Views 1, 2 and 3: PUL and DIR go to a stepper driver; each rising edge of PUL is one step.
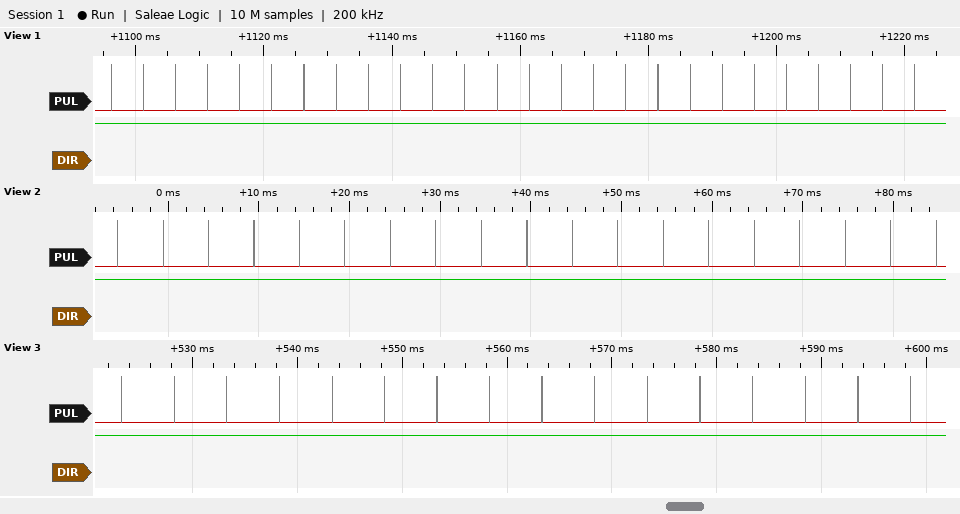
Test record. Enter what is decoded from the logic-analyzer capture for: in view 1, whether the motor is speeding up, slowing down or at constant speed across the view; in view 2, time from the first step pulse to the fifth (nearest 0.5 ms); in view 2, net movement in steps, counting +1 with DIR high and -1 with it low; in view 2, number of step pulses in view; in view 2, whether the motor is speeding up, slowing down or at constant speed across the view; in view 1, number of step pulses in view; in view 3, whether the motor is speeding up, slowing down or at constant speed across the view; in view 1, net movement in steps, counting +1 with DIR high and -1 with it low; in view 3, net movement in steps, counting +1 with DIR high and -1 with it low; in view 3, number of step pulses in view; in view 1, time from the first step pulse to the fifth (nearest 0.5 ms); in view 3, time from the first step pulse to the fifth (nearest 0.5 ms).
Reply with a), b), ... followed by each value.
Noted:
a) constant speed
b) 20.0 ms
c) +19
d) 19
e) constant speed
f) 26
g) constant speed
h) +26
i) +16
j) 16
k) 20.0 ms
l) 20.0 ms
